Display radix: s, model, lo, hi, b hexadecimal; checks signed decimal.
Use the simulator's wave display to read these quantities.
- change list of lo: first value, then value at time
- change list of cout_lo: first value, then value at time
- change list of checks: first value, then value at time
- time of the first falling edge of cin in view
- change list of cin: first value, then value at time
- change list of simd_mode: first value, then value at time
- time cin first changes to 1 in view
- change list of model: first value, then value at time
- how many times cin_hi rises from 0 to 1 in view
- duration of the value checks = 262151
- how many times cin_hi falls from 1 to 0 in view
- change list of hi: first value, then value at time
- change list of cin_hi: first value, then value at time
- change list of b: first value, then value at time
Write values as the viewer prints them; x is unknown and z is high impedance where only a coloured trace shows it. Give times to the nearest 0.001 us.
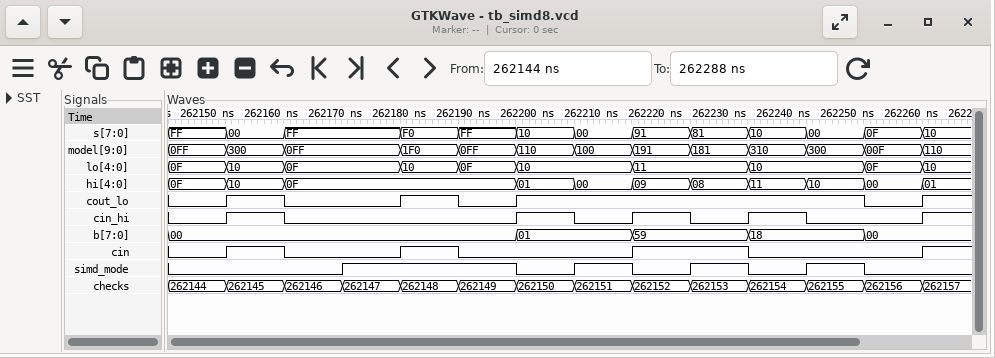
0F, 10 at 262.153 us, 0F at 262.162 us, 10 at 262.18 us, 0F at 262.189 us, 10 at 262.198 us, 11 at 262.216 us, 10 at 262.234 us, 0F at 262.252 us, 10 at 262.261 us
0, 1 at 262.153 us, 0 at 262.162 us, 1 at 262.18 us, 0 at 262.189 us, 1 at 262.198 us, 0 at 262.252 us, 1 at 262.261 us
262144, 262145 at 262.153 us, 262146 at 262.162 us, 262147 at 262.171 us, 262148 at 262.18 us, 262149 at 262.189 us, 262150 at 262.198 us, 262151 at 262.207 us, 262152 at 262.216 us, 262153 at 262.225 us, 262154 at 262.234 us, 262155 at 262.243 us, 262156 at 262.252 us, 262157 at 262.261 us
262.162 us
0, 1 at 262.153 us, 0 at 262.162 us, 1 at 262.18 us, 0 at 262.189 us, 1 at 262.216 us, 0 at 262.234 us, 1 at 262.261 us
0, 1 at 262.171 us, 0 at 262.198 us, 1 at 262.207 us, 0 at 262.216 us, 1 at 262.225 us, 0 at 262.234 us, 1 at 262.243 us, 0 at 262.252 us
262.153 us
0FF, 300 at 262.153 us, 0FF at 262.162 us, 1F0 at 262.18 us, 0FF at 262.189 us, 110 at 262.198 us, 100 at 262.207 us, 191 at 262.216 us, 181 at 262.225 us, 310 at 262.234 us, 300 at 262.243 us, 00F at 262.252 us, 110 at 262.261 us
5
0.009 us
4
0F, 10 at 262.153 us, 0F at 262.162 us, 01 at 262.198 us, 00 at 262.207 us, 09 at 262.216 us, 08 at 262.225 us, 11 at 262.234 us, 10 at 262.243 us, 00 at 262.252 us, 01 at 262.261 us
0, 1 at 262.153 us, 0 at 262.162 us, 1 at 262.198 us, 0 at 262.207 us, 1 at 262.216 us, 0 at 262.225 us, 1 at 262.234 us, 0 at 262.243 us, 1 at 262.261 us
00, 01 at 262.198 us, 59 at 262.216 us, 18 at 262.234 us, 00 at 262.252 us
